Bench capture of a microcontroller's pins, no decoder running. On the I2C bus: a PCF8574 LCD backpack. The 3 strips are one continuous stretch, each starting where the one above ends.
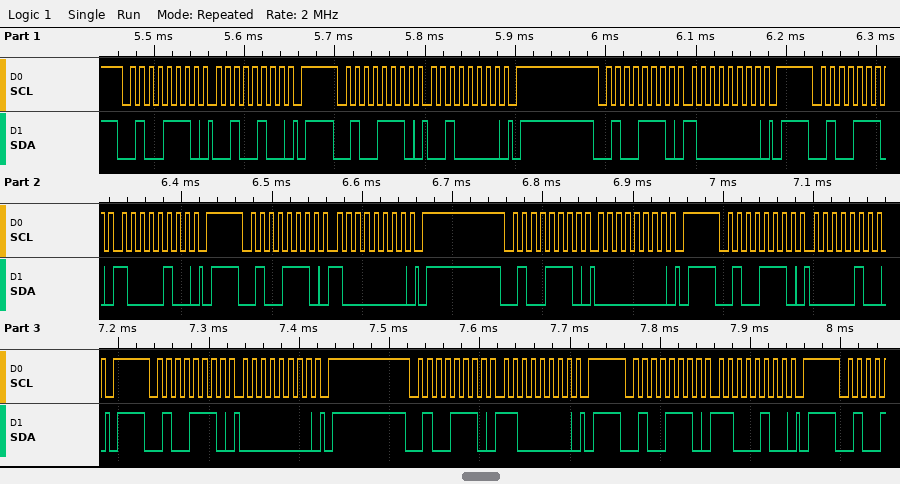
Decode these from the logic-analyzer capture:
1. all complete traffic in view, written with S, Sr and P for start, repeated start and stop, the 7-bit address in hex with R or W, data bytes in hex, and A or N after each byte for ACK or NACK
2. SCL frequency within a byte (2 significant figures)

S 27W A 24 A P S 27W A 20 A P S 27W A 80 A P S 27W A 84 A P S 27W A 80 A P S 27W A 00 A P S 27W A 04 A P S 27W A 00 A P S 27W A C0 A P S 27W A C4 A P
100 kHz
